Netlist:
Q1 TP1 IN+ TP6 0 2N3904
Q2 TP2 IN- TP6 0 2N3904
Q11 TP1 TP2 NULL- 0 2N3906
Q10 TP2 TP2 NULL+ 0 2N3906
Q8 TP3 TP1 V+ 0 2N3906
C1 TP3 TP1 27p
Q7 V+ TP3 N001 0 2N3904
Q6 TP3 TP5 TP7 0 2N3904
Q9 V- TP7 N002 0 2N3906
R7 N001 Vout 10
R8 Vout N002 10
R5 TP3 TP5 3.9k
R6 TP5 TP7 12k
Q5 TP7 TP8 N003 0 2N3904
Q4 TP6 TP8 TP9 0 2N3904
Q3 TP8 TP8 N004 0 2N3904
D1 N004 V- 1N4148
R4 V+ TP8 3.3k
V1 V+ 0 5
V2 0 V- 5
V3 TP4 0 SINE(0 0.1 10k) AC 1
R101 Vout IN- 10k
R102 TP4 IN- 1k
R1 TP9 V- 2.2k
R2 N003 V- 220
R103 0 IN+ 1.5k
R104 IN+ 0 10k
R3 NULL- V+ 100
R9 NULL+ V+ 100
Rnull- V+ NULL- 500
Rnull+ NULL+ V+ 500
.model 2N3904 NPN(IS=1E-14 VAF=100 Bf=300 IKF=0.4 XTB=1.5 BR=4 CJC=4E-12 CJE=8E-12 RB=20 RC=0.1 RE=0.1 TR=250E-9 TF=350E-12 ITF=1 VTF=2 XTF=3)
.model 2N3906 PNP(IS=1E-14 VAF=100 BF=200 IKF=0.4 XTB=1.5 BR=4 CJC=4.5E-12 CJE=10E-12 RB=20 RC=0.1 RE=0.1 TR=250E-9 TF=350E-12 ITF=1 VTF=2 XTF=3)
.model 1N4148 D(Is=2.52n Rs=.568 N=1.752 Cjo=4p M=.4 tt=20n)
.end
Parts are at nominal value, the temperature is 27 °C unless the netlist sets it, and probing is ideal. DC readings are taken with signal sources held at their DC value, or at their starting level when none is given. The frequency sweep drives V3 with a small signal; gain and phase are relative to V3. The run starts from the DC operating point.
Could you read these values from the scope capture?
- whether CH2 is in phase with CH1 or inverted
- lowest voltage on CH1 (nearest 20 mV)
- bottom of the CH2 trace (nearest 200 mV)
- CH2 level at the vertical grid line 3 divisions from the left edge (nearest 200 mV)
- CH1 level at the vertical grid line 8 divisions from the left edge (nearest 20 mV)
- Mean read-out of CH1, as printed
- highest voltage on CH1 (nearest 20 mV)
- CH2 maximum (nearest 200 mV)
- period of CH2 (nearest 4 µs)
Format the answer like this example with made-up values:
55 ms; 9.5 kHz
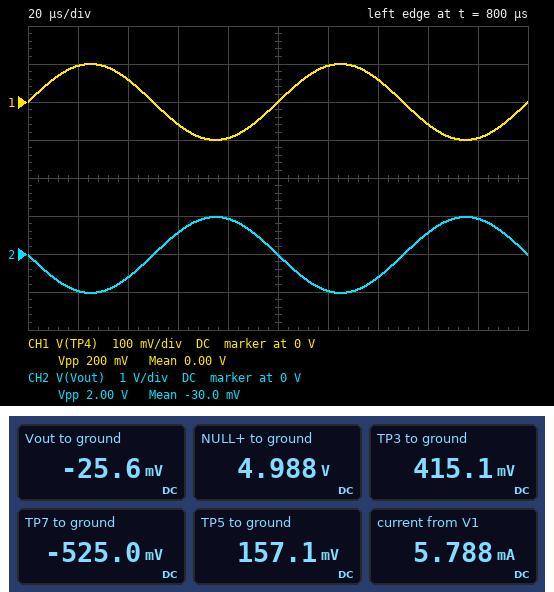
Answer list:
inverted; -100 mV; -1.0 V; 600 mV; -60 mV; 0.00 V; 100 mV; 1.0 V; 100 µs
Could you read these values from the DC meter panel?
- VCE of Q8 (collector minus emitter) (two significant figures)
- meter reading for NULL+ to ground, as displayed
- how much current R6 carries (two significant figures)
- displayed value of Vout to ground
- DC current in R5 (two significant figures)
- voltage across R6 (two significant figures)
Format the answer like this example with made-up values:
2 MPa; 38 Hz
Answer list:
-4.6 V; 4.988 V; 57 µA; -25.6 mV; 66 µA; 680 mV
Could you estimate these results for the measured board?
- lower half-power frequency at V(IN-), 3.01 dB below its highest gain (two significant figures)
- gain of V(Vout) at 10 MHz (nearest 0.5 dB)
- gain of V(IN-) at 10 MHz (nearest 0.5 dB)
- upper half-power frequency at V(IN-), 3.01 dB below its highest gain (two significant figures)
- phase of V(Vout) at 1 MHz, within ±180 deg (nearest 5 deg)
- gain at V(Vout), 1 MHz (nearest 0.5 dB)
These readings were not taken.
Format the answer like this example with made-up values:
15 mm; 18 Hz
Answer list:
2.5 MHz; 5.5 dB; -1.5 dB; 15 MHz; 155 deg; 18.5 dB
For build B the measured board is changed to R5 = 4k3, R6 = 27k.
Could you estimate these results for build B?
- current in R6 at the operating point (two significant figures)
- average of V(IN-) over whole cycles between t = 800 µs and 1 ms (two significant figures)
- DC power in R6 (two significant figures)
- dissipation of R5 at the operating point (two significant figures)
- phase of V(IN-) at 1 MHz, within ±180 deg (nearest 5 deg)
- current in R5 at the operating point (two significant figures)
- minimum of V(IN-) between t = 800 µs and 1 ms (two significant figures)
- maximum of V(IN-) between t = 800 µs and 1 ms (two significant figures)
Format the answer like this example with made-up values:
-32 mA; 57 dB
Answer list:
25 µA; -2.8 mV; 17 µW; 5.2 µW; 50 deg; 35 µA; -4.1 mV; -1.5 mV
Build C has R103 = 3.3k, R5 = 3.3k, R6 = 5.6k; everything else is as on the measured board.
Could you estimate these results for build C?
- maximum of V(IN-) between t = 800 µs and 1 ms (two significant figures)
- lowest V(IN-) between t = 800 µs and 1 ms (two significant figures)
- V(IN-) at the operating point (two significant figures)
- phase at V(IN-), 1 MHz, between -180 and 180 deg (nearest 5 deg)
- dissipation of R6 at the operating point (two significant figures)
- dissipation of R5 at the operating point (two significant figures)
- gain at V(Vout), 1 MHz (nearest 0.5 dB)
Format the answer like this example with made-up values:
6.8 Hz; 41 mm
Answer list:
-3.0 mV; -3.7 mV; -3.4 mV; 75 deg; 83 µW; 56 µW; 20.0 dB
